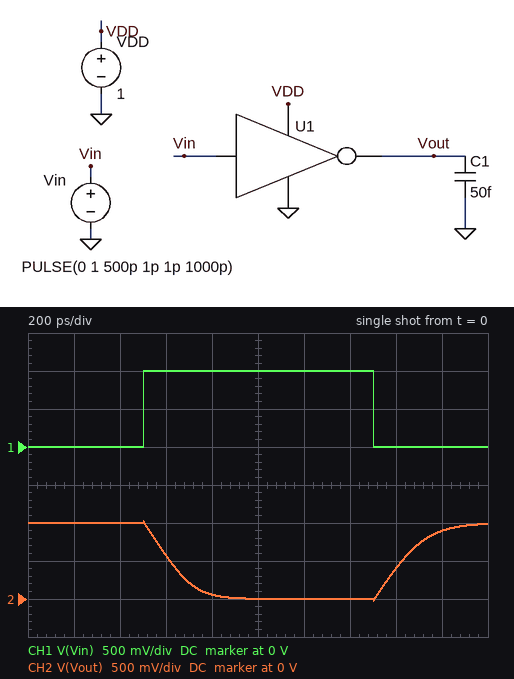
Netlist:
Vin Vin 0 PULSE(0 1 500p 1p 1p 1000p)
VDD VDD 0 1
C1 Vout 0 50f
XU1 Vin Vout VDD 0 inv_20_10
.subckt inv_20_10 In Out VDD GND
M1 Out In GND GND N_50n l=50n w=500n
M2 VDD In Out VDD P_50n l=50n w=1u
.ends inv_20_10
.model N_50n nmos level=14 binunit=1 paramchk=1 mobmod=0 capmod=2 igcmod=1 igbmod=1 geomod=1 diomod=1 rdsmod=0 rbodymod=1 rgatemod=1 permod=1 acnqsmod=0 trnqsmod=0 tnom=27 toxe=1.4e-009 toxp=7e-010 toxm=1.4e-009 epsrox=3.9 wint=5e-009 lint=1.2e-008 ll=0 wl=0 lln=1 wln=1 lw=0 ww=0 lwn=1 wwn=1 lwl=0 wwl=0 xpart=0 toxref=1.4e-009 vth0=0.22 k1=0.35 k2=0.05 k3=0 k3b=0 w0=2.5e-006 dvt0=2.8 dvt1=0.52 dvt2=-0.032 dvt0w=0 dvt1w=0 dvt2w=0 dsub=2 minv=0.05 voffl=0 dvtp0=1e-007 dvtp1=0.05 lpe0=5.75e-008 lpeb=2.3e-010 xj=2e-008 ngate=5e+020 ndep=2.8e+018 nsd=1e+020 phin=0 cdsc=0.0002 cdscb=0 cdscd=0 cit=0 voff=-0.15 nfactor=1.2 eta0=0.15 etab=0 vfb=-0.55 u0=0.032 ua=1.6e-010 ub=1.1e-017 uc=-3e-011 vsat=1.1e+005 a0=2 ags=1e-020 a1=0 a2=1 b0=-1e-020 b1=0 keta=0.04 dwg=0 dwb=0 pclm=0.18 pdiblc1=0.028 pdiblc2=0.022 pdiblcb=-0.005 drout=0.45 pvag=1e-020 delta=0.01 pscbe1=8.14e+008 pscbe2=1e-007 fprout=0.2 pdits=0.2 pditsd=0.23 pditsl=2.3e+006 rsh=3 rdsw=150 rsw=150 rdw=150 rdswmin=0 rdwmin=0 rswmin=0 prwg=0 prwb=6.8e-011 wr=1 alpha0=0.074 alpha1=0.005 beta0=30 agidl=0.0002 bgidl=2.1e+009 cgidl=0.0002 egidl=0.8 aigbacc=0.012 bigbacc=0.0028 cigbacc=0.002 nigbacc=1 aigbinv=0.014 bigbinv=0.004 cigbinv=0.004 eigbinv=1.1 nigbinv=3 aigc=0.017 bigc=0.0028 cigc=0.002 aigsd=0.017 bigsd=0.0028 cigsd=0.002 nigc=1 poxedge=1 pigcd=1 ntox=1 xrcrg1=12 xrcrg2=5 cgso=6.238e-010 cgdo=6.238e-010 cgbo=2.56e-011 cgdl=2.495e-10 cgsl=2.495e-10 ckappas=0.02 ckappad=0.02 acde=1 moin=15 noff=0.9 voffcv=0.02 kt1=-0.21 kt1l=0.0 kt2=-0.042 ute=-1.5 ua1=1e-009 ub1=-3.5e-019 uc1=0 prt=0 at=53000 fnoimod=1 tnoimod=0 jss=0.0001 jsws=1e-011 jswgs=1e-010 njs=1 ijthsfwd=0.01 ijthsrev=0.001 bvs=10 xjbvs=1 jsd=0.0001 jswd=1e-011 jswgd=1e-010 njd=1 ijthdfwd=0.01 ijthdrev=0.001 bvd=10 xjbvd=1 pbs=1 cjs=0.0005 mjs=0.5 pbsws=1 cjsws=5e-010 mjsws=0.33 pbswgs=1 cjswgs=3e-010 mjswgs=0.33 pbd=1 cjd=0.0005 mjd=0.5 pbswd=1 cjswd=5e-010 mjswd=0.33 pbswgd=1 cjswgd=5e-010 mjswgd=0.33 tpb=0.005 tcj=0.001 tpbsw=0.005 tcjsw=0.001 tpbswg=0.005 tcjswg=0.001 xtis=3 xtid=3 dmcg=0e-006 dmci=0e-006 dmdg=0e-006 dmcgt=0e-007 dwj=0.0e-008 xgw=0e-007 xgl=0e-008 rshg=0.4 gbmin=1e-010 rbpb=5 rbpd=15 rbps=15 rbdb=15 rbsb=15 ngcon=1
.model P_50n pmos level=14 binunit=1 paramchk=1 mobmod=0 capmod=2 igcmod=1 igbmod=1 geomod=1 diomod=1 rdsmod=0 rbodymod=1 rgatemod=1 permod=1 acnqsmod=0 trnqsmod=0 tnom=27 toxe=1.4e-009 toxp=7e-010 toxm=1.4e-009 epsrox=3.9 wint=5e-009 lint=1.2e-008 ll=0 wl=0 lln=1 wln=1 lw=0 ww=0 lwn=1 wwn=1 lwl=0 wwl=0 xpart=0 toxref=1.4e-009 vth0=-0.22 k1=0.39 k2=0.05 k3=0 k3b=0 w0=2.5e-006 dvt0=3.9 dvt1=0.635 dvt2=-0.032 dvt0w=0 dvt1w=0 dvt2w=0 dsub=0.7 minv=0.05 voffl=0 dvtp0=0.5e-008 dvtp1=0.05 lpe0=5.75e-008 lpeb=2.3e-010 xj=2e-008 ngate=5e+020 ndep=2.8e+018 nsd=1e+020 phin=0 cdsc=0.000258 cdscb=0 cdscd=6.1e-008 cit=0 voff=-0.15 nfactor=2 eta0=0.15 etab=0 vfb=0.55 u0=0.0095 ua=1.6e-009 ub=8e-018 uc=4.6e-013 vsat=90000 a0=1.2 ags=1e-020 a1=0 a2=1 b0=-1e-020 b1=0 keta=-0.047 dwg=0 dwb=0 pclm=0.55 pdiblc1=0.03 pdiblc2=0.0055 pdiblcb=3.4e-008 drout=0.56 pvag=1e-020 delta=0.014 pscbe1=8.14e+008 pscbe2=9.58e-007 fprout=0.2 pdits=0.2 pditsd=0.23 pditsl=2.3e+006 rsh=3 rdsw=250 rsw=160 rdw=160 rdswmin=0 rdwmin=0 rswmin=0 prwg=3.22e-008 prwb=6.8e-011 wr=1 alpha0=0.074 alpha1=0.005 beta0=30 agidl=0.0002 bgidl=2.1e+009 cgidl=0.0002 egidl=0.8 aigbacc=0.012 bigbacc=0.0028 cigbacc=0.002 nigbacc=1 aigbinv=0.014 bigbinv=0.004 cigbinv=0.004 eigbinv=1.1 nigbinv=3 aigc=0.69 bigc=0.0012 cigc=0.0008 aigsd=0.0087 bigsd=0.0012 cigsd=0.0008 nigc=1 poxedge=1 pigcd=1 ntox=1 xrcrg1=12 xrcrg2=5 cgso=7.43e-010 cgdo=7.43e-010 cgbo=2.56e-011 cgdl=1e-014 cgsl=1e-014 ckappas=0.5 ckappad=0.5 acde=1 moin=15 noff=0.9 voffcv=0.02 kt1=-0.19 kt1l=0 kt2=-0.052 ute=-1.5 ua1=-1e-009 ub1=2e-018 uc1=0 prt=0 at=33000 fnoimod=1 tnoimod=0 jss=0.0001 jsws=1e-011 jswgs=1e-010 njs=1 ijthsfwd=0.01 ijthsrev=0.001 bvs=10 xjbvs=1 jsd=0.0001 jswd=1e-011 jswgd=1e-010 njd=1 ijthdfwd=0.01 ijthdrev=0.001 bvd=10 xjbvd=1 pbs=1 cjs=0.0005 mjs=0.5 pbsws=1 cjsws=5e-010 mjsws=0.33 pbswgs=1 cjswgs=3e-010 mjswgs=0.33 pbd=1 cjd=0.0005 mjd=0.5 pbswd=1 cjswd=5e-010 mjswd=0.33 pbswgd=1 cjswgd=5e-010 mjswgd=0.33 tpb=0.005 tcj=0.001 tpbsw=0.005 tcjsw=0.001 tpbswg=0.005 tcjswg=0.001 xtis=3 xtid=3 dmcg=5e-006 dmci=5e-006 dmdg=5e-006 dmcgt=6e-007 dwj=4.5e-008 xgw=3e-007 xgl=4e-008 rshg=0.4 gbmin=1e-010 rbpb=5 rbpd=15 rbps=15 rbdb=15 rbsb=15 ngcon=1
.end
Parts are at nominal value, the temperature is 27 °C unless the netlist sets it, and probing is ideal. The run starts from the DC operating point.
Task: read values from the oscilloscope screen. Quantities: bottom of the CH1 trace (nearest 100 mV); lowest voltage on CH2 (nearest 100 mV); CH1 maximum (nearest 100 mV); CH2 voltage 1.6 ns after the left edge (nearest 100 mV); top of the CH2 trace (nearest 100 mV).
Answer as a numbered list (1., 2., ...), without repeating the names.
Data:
1. 0 V
2. 0 V
3. 1.0 V
4. 400 mV
5. 1.0 V
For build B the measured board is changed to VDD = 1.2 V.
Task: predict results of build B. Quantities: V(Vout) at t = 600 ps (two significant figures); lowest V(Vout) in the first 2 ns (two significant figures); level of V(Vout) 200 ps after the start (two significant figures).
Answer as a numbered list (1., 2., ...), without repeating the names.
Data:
1. 750 mV
2. -23 mV
3. 1.2 V
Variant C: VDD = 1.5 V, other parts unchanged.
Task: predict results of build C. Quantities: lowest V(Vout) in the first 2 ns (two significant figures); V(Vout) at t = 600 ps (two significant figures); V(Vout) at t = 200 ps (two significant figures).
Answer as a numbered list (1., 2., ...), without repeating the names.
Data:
1. 78 mV
2. 1.1 V
3. 1.5 V
